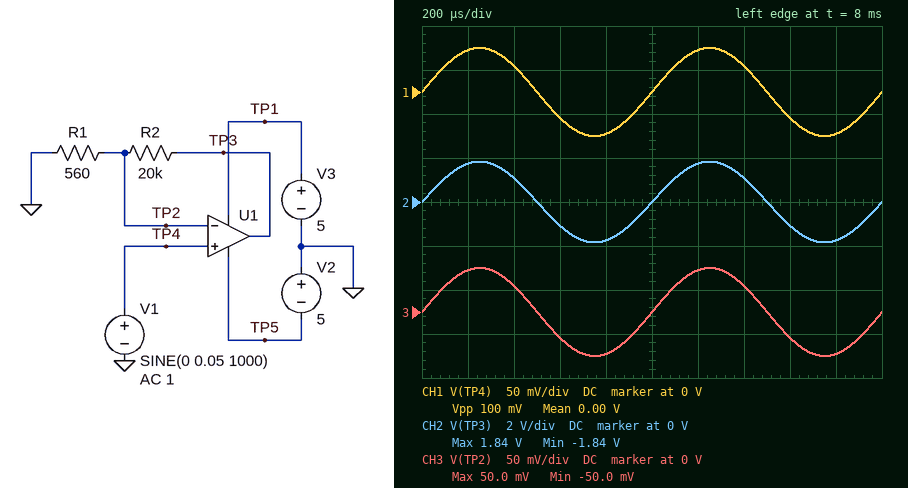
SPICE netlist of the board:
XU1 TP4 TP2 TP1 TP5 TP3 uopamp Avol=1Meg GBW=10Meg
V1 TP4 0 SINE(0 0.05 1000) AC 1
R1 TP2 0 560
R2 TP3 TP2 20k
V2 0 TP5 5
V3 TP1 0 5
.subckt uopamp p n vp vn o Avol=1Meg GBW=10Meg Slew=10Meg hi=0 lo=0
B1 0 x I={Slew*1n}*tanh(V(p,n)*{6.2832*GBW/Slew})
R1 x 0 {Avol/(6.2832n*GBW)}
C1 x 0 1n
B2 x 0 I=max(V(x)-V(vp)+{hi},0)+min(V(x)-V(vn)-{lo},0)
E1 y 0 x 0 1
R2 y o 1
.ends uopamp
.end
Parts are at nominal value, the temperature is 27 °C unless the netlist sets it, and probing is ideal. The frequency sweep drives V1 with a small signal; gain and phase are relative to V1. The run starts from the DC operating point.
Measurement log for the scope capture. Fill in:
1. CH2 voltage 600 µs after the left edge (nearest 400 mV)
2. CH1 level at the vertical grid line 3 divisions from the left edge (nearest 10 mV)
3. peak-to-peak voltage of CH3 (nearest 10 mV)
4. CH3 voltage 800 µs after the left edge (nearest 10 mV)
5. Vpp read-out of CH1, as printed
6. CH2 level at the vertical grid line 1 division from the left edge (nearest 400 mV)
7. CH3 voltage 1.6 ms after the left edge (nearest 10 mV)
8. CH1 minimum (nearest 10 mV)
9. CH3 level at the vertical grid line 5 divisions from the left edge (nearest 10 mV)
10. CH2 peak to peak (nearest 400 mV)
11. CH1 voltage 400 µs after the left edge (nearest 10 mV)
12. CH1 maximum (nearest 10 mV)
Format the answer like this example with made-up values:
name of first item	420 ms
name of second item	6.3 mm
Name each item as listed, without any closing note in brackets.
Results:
CH2 voltage 600 µs after the left edge	-1.2 V
CH1 level at the vertical grid line 3 divisions from the left edge	-30 mV
peak-to-peak voltage of CH3	100 mV
CH3 voltage 800 µs after the left edge	-50 mV
Vpp read-out of CH1, as printed	100 mV
CH2 level at the vertical grid line 1 division from the left edge	1.6 V
CH3 voltage 1.6 ms after the left edge	-30 mV
CH1 minimum	-50 mV
CH3 level at the vertical grid line 5 divisions from the left edge	0 V
CH2 peak to peak	3.6 V
CH1 voltage 400 µs after the left edge	30 mV
CH1 maximum	50 mV
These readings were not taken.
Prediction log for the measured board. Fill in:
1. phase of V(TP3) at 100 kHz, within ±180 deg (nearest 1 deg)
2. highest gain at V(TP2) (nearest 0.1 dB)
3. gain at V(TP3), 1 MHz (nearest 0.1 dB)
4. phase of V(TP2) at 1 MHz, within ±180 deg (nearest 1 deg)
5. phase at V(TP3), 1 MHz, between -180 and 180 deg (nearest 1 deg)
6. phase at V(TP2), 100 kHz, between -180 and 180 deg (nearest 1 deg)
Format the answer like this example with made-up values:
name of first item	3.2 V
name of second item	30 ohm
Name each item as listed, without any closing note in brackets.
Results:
phase of V(TP3) at 100 kHz, within ±180 deg	-20 deg
highest gain at V(TP2)	0 dB
gain at V(TP3), 1 MHz	19.7 dB
phase of V(TP2) at 1 MHz, within ±180 deg	-75 deg
phase at V(TP3), 1 MHz, between -180 and 180 deg	-75 deg
phase at V(TP2), 100 kHz, between -180 and 180 deg	-20 deg
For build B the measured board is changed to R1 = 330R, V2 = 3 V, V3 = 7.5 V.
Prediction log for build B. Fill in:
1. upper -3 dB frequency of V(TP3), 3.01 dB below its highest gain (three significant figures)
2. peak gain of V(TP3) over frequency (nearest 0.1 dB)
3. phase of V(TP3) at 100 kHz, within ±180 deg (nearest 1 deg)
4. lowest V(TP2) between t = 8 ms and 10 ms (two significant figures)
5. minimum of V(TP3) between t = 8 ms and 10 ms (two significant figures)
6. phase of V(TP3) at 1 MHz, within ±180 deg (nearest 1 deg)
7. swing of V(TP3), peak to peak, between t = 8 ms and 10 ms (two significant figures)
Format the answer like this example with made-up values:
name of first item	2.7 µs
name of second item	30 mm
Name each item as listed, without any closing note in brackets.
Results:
upper -3 dB frequency of V(TP3), 3.01 dB below its highest gain	162 kHz
peak gain of V(TP3) over frequency	35.8 dB
phase of V(TP3) at 100 kHz, within ±180 deg	-32 deg
lowest V(TP2) between t = 8 ms and 10 ms	-49 mV
minimum of V(TP3) between t = 8 ms and 10 ms	-3.0 V
phase of V(TP3) at 1 MHz, within ±180 deg	-81 deg
swing of V(TP3), peak to peak, between t = 8 ms and 10 ms	6.1 V
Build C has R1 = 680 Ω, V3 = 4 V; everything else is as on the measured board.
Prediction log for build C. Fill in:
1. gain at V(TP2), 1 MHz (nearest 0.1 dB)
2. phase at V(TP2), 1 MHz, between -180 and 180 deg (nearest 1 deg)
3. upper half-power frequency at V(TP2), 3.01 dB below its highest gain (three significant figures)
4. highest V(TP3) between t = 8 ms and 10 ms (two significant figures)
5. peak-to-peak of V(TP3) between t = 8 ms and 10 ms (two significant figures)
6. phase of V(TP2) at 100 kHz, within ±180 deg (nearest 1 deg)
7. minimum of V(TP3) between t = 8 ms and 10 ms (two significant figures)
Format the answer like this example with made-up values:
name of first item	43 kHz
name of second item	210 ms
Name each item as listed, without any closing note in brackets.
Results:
gain at V(TP2), 1 MHz	-10.1 dB
phase at V(TP2), 1 MHz, between -180 and 180 deg	-72 deg
upper half-power frequency at V(TP2), 3.01 dB below its highest gain	329 kHz
highest V(TP3) between t = 8 ms and 10 ms	1.5 V
peak-to-peak of V(TP3) between t = 8 ms and 10 ms	3.0 V
phase of V(TP2) at 100 kHz, within ±180 deg	-17 deg
minimum of V(TP3) between t = 8 ms and 10 ms	-1.5 V
